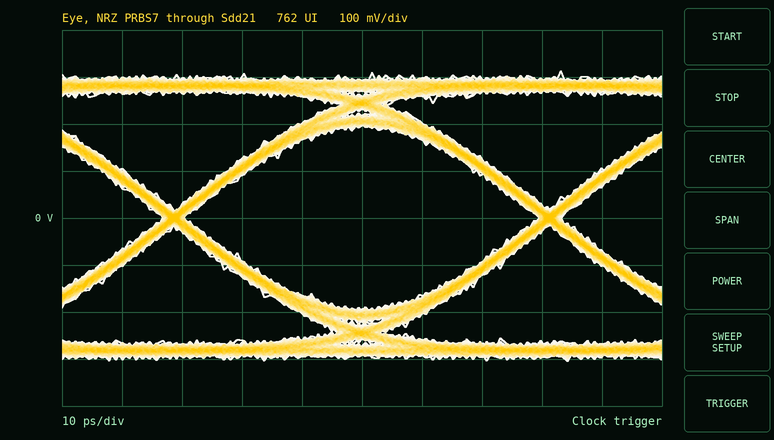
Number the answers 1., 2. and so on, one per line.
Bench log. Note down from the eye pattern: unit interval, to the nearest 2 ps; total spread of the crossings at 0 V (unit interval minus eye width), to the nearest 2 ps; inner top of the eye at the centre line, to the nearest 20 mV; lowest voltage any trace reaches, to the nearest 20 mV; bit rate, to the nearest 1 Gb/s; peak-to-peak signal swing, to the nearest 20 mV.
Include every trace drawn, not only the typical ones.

1. 62 ps
2. 4 ps
3. 200 mV
4. -300 mV
5. 16 Gb/s
6. 620 mV
